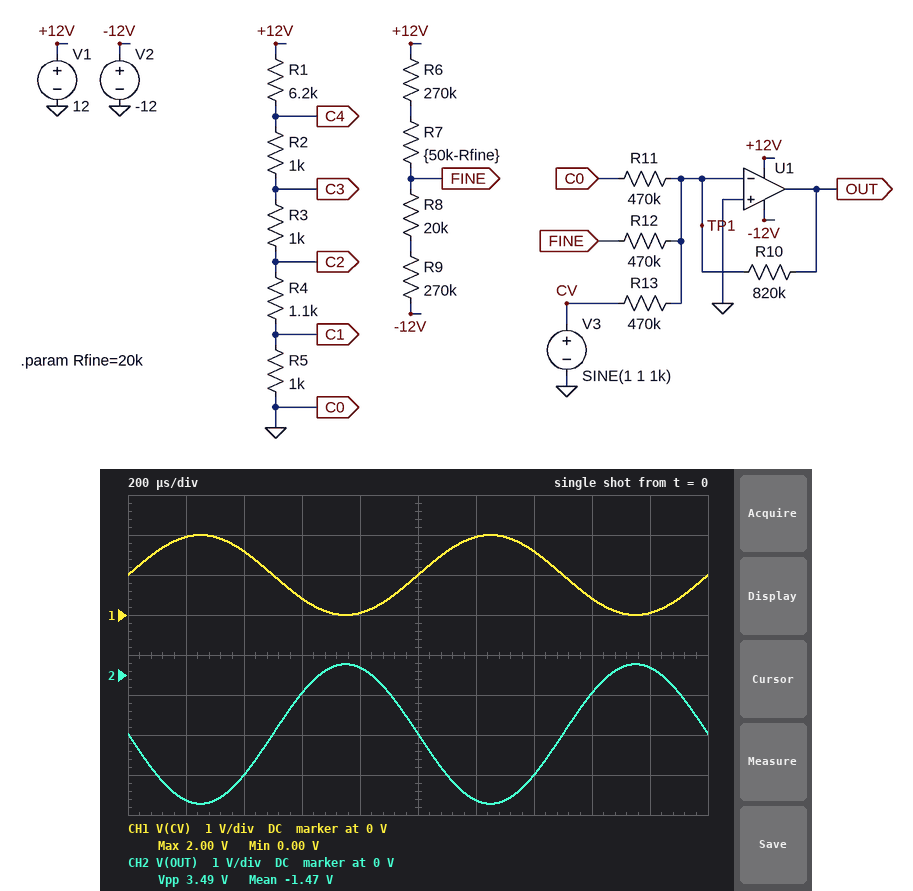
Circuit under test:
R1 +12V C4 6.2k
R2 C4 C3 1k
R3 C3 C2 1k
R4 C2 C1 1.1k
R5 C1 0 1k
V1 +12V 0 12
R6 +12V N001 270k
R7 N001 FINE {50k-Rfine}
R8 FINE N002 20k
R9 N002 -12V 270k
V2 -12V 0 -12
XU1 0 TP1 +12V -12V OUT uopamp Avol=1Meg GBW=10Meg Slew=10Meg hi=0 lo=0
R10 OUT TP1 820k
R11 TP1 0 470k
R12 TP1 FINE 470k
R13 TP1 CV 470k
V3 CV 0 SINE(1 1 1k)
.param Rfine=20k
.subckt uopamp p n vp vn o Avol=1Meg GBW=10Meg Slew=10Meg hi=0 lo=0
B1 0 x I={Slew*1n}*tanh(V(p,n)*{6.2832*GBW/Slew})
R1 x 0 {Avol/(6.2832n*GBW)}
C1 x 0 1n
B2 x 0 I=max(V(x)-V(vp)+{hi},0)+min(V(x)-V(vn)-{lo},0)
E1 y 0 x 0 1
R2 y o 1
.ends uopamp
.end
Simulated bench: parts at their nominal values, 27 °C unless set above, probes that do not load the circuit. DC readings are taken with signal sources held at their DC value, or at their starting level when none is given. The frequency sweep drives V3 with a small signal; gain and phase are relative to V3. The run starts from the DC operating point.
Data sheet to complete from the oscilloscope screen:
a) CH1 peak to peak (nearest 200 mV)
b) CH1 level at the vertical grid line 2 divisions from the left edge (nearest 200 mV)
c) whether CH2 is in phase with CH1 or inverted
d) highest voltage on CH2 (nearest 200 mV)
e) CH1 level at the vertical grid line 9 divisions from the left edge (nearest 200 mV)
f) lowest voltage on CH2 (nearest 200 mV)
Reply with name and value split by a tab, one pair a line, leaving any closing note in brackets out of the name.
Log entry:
CH1 peak to peak	2.0 V
CH1 level at the vertical grid line 2 divisions from the left edge	1.6 V
whether CH2 is in phase with CH1 or inverted	inverted
highest voltage on CH2	200 mV
CH1 level at the vertical grid line 9 divisions from the left edge	0 V
lowest voltage on CH2	-3.2 V
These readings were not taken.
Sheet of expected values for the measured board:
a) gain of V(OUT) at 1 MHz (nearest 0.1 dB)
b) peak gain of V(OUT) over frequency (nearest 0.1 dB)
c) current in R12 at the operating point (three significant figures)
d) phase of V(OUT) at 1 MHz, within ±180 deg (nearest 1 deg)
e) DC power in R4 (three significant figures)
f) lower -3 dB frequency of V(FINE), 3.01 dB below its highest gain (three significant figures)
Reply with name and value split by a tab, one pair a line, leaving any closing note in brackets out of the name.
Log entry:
gain of V(OUT) at 1 MHz	3.6 dB
peak gain of V(OUT) over frequency	4.8 dB
current in R12 at the operating point	329 nA
phase of V(OUT) at 1 MHz, within ±180 deg	150 deg
DC power in R4	1.49 mW
lower -3 dB frequency of V(FINE), 3.01 dB below its highest gain	1.72 MHz
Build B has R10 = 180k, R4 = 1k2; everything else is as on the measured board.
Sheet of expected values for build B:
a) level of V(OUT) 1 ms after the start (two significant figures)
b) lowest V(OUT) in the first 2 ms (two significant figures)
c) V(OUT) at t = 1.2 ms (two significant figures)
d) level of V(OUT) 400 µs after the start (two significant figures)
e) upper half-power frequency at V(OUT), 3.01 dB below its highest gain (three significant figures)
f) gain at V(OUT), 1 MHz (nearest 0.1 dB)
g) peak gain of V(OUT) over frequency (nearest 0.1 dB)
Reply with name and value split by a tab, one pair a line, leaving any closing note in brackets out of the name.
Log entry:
level of V(OUT) 1 ms after the start	-320 mV
lowest V(OUT) in the first 2 ms	-710 mV
V(OUT) at t = 1.2 ms	-690 mV
level of V(OUT) 400 µs after the start	-550 mV
upper half-power frequency at V(OUT), 3.01 dB below its highest gain	4.86 MHz
gain at V(OUT), 1 MHz	-8.5 dB
peak gain of V(OUT) over frequency	-8.3 dB
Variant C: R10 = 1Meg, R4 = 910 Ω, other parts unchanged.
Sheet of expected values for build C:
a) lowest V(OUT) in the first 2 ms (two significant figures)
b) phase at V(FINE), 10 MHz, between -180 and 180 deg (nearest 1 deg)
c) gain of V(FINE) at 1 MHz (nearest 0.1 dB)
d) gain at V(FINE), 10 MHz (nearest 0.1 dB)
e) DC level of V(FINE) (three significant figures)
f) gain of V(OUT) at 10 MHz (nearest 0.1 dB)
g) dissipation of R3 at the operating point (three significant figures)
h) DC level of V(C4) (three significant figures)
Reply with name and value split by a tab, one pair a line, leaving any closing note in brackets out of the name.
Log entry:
lowest V(OUT) in the first 2 ms	-3.9 V
phase at V(FINE), 10 MHz, between -180 and 180 deg	8 deg
gain of V(FINE) at 1 MHz	-27.6 dB
gain at V(FINE), 10 MHz	-22.7 dB
DC level of V(FINE)	-155 mV
gain of V(OUT) at 10 MHz	-10.3 dB
dissipation of R3 at the operating point	1.41 mW
DC level of V(C4)	4.64 V
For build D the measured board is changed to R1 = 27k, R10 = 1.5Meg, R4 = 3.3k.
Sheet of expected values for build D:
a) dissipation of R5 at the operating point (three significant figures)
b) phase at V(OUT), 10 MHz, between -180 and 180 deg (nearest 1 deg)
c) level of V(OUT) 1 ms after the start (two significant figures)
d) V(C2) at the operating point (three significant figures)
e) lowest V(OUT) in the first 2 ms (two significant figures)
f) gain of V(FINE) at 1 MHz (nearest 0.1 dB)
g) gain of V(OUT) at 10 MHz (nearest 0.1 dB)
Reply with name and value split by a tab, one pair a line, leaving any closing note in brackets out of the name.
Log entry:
dissipation of R5 at the operating point	130 µW
phase at V(OUT), 10 MHz, between -180 and 180 deg	96 deg
level of V(OUT) 1 ms after the start	-2.7 V
V(C2) at the operating point	1.55 V
lowest V(OUT) in the first 2 ms	-5.9 V
gain of V(FINE) at 1 MHz	-25.3 dB
gain of V(OUT) at 10 MHz	-9.8 dB
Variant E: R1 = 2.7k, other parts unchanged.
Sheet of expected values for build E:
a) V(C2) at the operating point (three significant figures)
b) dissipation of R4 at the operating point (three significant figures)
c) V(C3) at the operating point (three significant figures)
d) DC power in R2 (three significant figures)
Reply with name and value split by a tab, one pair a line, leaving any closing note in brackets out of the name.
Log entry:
V(C2) at the operating point	3.71 V
dissipation of R4 at the operating point	3.43 mW
V(C3) at the operating point	5.47 V
DC power in R2	3.11 mW
